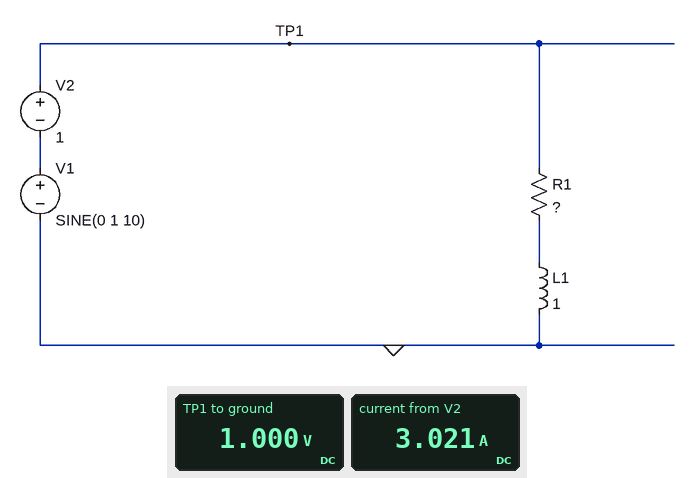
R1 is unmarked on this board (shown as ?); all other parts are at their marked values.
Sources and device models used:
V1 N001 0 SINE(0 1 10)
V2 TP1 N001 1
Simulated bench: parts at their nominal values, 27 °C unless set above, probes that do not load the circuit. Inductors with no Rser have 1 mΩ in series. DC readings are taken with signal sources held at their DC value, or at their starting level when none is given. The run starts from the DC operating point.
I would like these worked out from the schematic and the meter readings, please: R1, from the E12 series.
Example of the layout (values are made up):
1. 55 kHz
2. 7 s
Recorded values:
1. 0.33 Ω
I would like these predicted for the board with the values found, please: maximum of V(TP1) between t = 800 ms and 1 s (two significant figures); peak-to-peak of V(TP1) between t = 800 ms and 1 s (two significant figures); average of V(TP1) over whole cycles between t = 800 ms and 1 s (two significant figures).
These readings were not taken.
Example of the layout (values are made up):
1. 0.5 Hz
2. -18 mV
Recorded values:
1. 2.0 V
2. 2.0 V
3. 1.0 V
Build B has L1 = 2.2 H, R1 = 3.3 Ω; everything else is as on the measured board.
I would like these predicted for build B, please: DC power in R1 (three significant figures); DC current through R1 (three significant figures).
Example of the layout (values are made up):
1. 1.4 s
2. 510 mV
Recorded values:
1. 303 mW
2. 303 mA
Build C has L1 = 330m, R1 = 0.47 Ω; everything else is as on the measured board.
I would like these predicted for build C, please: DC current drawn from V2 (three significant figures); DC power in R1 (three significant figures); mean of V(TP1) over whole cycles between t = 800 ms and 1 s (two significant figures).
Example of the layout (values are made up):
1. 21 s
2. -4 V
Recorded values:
1. 2.12 A
2. 2.12 W
3. 1.0 V
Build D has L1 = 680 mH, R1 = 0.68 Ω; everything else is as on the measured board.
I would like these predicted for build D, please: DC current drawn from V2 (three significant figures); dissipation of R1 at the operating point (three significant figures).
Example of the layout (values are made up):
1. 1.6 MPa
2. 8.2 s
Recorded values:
1. 1.47 A
2. 1.47 W
